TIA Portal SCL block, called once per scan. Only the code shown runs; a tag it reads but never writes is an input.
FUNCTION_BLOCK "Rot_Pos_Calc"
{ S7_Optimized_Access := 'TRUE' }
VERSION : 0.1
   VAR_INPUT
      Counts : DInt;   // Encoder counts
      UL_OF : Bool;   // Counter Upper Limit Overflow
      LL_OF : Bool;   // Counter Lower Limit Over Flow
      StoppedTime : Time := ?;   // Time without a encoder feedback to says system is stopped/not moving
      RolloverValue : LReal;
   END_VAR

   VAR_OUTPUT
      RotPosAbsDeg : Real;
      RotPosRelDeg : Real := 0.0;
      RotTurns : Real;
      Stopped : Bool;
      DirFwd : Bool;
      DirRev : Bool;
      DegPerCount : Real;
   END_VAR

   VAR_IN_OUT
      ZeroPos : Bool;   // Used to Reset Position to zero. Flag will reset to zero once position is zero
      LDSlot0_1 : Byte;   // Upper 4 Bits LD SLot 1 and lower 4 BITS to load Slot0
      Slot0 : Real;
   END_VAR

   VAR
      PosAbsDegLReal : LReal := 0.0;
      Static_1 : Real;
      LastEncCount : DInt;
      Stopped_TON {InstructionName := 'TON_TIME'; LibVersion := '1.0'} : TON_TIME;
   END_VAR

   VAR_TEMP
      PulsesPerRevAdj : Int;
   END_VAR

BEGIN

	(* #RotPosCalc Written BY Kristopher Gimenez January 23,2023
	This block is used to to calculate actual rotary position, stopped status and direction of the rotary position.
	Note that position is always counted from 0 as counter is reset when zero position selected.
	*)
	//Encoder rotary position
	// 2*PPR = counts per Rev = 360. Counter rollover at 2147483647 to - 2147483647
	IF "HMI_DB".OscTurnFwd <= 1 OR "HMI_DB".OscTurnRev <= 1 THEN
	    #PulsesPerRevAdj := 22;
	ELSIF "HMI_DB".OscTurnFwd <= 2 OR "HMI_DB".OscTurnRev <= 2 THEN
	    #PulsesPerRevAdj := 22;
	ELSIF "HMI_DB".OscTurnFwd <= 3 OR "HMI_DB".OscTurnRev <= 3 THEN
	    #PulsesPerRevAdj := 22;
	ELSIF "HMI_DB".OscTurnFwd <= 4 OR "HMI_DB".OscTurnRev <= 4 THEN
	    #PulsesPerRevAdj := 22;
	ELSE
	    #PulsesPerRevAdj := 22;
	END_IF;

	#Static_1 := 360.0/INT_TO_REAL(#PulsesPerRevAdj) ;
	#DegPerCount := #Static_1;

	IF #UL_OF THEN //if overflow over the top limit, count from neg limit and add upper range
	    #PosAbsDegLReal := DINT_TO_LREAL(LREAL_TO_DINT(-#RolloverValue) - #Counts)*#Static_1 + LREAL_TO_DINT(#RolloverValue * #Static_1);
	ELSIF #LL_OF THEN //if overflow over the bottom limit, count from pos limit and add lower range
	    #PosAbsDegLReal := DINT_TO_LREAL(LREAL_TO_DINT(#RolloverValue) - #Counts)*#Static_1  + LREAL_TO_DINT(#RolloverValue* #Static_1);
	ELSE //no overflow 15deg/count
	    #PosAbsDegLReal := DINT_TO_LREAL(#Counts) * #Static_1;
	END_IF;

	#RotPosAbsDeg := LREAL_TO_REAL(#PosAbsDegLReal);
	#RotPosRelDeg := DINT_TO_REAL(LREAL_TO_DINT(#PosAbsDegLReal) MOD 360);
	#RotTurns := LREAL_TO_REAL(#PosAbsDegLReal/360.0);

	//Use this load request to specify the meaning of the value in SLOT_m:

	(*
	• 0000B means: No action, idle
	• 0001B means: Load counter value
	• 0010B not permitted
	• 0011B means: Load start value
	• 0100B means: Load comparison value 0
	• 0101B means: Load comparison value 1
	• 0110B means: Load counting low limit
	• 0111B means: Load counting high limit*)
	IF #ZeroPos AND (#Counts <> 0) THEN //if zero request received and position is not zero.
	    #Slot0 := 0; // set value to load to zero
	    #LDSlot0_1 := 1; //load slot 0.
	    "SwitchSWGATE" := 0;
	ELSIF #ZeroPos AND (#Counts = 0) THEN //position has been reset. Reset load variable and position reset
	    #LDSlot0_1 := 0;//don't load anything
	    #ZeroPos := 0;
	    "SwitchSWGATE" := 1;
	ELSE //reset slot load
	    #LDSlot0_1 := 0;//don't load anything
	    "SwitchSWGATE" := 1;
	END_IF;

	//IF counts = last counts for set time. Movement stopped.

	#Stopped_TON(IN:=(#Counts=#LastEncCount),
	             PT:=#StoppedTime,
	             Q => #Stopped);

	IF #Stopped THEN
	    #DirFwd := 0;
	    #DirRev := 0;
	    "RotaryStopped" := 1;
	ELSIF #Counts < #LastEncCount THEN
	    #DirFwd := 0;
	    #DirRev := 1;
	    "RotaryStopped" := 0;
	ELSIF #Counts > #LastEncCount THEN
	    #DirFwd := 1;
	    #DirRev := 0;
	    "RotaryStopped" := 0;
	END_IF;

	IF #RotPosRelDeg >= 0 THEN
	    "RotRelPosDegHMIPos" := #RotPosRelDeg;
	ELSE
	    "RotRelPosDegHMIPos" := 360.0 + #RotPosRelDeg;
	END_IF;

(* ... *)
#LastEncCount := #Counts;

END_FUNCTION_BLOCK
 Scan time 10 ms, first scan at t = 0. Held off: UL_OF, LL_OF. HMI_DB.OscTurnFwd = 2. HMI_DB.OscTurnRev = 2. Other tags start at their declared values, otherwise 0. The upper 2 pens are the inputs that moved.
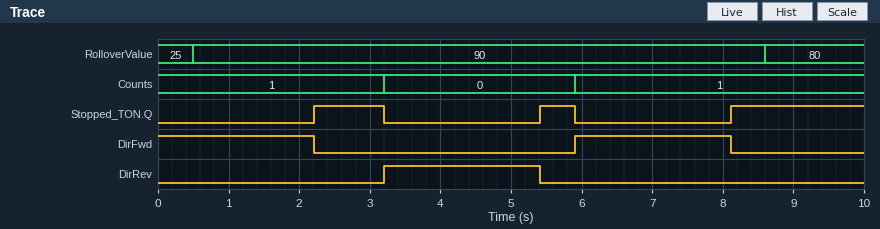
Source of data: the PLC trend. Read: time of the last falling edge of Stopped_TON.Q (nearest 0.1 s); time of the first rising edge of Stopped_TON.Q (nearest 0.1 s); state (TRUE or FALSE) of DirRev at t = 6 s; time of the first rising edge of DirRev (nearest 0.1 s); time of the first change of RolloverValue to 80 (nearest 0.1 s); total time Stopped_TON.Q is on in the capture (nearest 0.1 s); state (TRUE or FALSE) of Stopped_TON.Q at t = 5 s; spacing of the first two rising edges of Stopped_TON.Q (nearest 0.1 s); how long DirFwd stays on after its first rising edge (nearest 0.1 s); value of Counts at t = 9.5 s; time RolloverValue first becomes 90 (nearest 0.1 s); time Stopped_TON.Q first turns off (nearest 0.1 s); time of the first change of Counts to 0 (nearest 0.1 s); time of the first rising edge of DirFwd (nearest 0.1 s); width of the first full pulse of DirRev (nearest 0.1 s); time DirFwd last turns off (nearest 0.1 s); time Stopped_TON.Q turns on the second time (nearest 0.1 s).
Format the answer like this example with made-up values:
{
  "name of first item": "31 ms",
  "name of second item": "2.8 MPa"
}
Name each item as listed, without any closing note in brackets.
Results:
{
  "time of the last falling edge of Stopped_TON.Q": "5.9 s",
  "time of the first rising edge of Stopped_TON.Q": "2.2 s",
  "state (TRUE or FALSE) of DirRev at t = 6 s": "FALSE",
  "time of the first rising edge of DirRev": "3.2 s",
  "time of the first change of RolloverValue to 80": "8.6 s",
  "total time Stopped_TON.Q is on in the capture": "3.4 s",
  "state (TRUE or FALSE) of Stopped_TON.Q at t = 5 s": "FALSE",
  "spacing of the first two rising edges of Stopped_TON.Q": "3.2 s",
  "how long DirFwd stays on after its first rising edge": "2.2 s",
  "value of Counts at t = 9.5 s": "1",
  "time RolloverValue first becomes 90": "0.5 s",
  "time Stopped_TON.Q first turns off": "3.2 s",
  "time of the first change of Counts to 0": "3.2 s",
  "time of the first rising edge of DirFwd": "5.9 s",
  "width of the first full pulse of DirRev": "2.2 s",
  "time DirFwd last turns off": "8.1 s",
  "time Stopped_TON.Q turns on the second time": "5.4 s"
}
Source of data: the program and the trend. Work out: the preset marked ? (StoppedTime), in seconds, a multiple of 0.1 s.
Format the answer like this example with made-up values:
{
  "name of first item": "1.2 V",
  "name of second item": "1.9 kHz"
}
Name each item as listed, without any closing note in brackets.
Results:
{
  "the preset marked ? (StoppedTime), in seconds, a multiple of 0.1 s": "2.2 s"
}
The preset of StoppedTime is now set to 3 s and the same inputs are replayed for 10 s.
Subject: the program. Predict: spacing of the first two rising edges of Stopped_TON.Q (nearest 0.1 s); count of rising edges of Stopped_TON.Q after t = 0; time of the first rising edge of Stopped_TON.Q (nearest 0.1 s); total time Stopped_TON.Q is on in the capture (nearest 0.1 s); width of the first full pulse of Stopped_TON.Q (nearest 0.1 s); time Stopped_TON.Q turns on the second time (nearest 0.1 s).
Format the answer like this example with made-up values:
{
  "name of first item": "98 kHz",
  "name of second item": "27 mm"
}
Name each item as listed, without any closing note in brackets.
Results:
{
  "spacing of the first two rising edges of Stopped_TON.Q": "5.9 s",
  "count of rising edges of Stopped_TON.Q after t = 0": "2",
  "time of the first rising edge of Stopped_TON.Q": "3.0 s",
  "total time Stopped_TON.Q is on in the capture": "1.3 s",
  "width of the first full pulse of Stopped_TON.Q": "0.2 s",
  "time Stopped_TON.Q turns on the second time": "8.9 s"
}
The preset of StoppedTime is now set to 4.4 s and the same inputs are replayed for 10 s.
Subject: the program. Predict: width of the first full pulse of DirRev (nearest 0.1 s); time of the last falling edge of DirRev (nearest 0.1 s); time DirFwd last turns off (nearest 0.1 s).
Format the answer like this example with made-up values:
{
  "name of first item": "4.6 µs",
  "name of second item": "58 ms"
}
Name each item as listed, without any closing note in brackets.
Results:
{
  "width of the first full pulse of DirRev": "2.7 s",
  "time of the last falling edge of DirRev": "5.9 s",
  "time DirFwd last turns off": "3.2 s"
}
